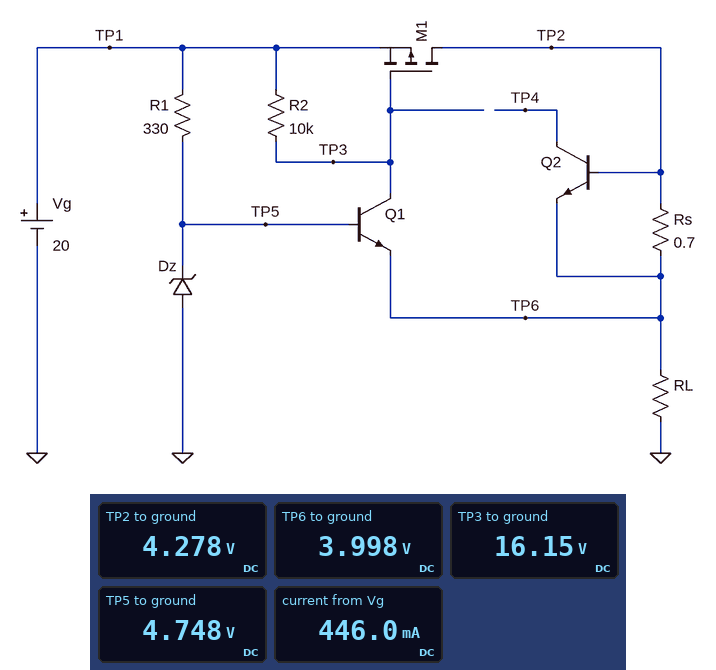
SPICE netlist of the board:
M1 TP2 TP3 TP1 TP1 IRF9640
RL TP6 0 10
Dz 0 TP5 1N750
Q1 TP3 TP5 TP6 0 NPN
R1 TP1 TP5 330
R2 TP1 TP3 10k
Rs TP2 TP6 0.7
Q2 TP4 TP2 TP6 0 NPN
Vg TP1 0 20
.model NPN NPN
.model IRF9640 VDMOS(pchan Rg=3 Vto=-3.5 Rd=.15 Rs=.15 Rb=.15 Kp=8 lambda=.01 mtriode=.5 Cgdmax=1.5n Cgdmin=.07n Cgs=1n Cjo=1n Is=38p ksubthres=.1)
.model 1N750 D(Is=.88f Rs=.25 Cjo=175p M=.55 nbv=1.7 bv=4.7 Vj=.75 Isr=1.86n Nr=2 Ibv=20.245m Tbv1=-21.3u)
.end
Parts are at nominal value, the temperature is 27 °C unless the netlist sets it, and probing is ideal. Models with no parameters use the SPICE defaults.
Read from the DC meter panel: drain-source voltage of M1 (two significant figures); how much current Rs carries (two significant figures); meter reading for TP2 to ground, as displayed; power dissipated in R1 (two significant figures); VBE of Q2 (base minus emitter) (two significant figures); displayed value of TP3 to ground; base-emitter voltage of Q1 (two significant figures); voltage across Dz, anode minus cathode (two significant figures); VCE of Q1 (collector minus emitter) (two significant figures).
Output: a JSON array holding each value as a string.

["-16 V", "400 mA", "4.278 V", "700 mW", "280 mV", "16.15 V", "750 mV", "-4.7 V", "12 V"]
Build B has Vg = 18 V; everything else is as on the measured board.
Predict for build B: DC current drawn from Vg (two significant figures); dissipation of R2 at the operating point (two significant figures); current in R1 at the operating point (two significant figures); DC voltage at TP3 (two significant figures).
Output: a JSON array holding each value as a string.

["440 mA", "1.5 mW", "40 mA", "14 V"]
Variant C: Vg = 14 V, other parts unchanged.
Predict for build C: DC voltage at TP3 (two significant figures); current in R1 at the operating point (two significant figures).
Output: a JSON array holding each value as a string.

["10 V", "28 mA"]
